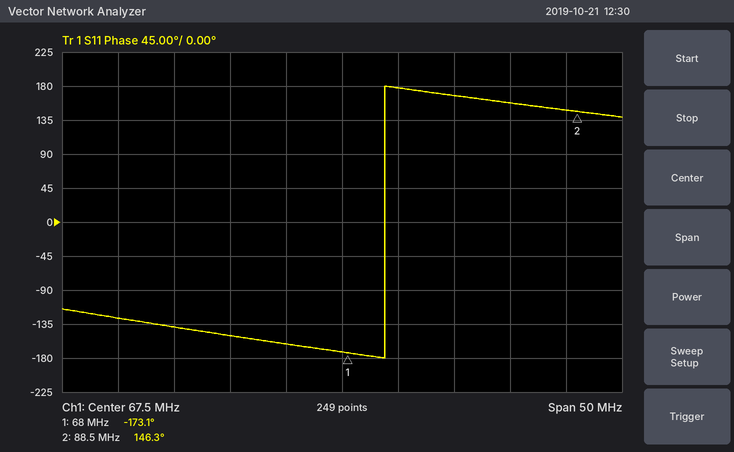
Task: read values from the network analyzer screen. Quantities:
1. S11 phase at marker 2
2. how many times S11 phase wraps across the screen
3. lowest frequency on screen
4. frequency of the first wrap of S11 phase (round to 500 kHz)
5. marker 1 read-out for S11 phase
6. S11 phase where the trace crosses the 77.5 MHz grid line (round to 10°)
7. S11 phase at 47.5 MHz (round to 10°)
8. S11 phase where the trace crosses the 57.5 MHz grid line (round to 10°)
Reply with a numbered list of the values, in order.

1. 146.3°
2. 1
3. 42.5 MHz
4. 71.5 MHz
5. -173.1°
6. 170°
7. -130°
8. -150°
